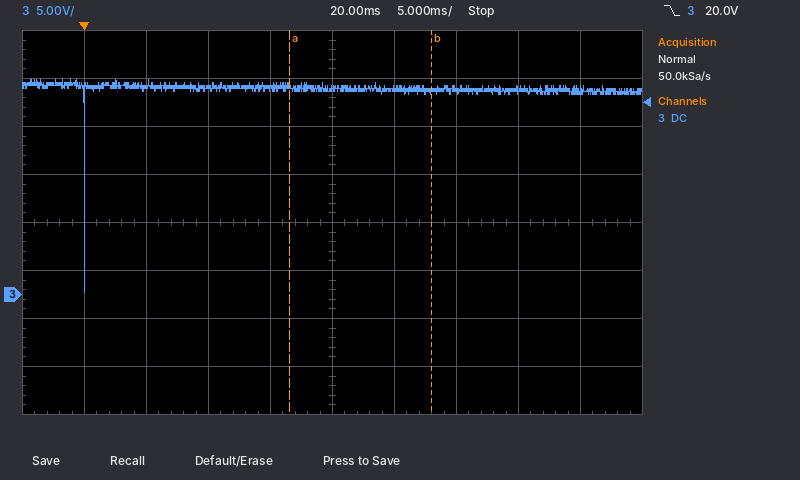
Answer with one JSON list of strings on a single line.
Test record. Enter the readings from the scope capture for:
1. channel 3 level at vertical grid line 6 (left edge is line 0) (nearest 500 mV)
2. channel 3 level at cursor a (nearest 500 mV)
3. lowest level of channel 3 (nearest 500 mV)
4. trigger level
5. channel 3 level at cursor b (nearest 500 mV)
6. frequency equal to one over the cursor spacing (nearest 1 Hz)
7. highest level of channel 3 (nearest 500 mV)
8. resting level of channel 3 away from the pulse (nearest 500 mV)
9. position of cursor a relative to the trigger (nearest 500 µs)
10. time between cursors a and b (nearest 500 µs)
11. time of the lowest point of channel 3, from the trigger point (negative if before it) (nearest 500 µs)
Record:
["21.5 V", "21.5 V", "0.0 V", "20.0 V", "21.0 V", "87 Hz", "22.5 V", "21.5 V", "+16.5 ms", "11.5 ms", "0.0 ms"]
